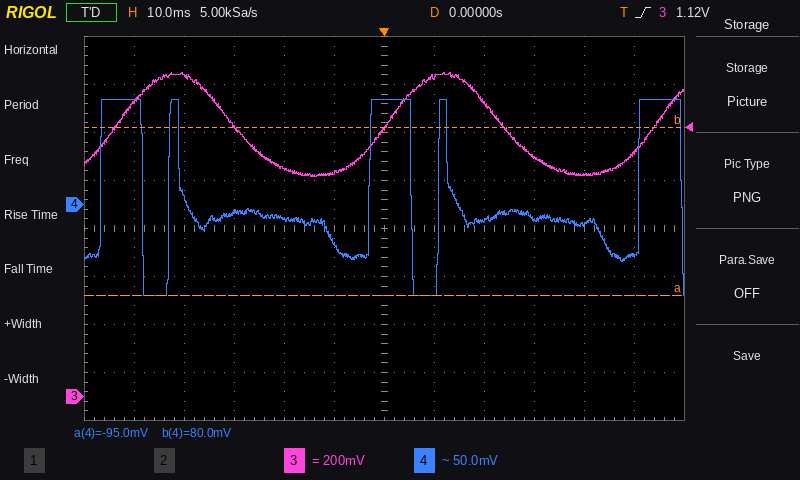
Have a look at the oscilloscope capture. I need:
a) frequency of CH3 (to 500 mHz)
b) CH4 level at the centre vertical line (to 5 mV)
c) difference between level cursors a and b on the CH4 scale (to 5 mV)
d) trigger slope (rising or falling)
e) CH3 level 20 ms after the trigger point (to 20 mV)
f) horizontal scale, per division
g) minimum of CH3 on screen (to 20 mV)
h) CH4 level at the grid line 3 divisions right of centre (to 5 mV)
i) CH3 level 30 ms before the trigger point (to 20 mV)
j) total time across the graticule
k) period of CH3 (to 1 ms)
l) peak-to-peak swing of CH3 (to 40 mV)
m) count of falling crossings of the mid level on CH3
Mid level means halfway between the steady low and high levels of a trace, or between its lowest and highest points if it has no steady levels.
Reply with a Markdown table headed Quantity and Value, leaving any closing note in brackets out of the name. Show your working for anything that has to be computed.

| Quantity | Value |
|---|---|
| frequency of CH3 | 1 / 54 ms ≈ 18.5 Hz |
| CH4 level at the centre vertical line | 110 mV |
| difference between level cursors a and b on the CH4 scale | 175 mV |
| trigger slope | rising |
| CH3 level 20 ms after the trigger point | 1.22 V |
| horizontal scale, per division | 10 ms |
| minimum of CH3 on screen | 920 mV |
| CH4 level at the grid line 3 divisions right of centre | -15 mV |
| CH3 level 30 ms before the trigger point | 1.12 V |
| total time across the graticule | 120 ms |
| period of CH3 | 54 ms |
| peak-to-peak swing of CH3 | 440 mV |
| count of falling crossings of the mid level on CH3 | 2 |
